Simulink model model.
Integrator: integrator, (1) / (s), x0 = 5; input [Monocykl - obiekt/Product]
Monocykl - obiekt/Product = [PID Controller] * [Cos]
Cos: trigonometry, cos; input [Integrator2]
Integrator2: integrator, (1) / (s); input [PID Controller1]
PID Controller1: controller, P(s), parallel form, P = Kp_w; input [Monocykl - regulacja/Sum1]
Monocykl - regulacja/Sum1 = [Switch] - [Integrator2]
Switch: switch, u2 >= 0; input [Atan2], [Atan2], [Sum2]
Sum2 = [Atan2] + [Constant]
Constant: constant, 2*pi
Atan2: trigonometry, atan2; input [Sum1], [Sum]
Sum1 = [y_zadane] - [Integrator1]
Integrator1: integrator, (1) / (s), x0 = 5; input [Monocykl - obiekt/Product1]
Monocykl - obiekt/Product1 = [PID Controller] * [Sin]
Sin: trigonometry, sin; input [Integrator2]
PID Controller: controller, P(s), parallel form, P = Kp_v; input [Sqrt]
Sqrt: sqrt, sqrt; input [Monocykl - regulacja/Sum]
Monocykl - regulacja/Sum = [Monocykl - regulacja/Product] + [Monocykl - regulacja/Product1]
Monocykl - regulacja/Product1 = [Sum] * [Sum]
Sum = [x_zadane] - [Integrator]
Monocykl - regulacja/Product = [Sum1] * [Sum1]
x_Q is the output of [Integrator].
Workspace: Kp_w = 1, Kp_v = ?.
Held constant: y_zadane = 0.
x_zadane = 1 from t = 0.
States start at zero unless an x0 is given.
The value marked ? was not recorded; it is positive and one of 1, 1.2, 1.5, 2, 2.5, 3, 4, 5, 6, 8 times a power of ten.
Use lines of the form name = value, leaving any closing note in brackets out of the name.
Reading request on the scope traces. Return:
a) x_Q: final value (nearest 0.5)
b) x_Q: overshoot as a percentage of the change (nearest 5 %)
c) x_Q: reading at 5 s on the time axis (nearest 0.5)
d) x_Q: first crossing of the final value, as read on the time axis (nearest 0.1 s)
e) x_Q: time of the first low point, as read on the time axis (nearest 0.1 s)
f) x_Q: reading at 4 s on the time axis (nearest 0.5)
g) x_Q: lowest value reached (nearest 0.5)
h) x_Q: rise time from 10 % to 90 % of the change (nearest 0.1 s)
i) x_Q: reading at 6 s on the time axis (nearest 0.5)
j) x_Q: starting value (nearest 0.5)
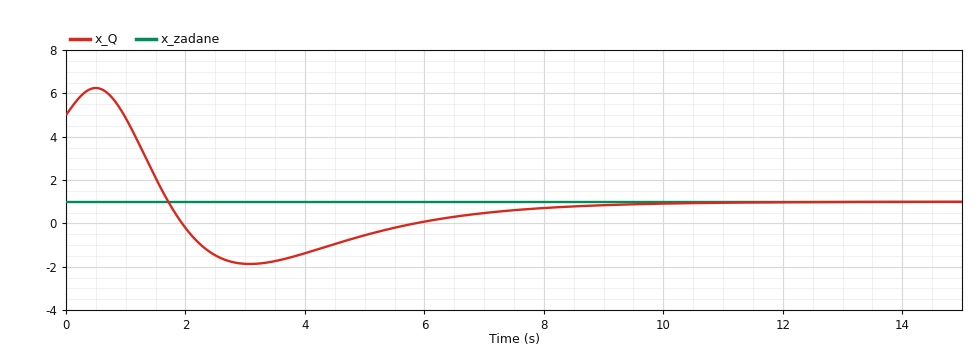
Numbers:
x_Q: final value = 1.0
x_Q: overshoot as a percentage of the change = 70 %
x_Q: reading at 5 s on the time axis = -0.5
x_Q: first crossing of the final value, as read on the time axis = 1.7 s
x_Q: time of the first low point, as read on the time axis = 3.1 s
x_Q: reading at 4 s on the time axis = -1.5
x_Q: lowest value reached = -2.0
x_Q: rise time from 10 % to 90 % of the change = 0.6 s
x_Q: reading at 6 s on the time axis = 0.0
x_Q: starting value = 5.0
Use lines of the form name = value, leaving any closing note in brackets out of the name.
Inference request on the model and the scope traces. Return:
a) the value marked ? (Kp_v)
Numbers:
the value marked ? = 0.6
